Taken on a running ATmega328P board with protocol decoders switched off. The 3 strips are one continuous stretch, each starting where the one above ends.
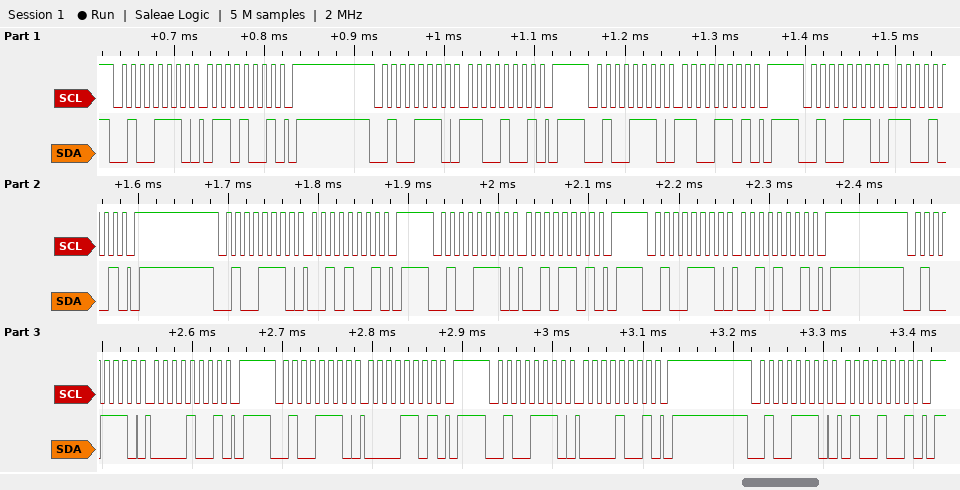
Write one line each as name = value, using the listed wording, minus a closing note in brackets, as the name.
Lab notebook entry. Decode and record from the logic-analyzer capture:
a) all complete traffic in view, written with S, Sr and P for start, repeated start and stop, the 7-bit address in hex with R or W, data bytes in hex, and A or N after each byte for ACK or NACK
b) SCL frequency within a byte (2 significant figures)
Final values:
all complete traffic in view, written with S, Sr and P for start, repeated start and stop, the 7-bit address in hex with R or W, data bytes in hex, and A or N after each byte for ACK or NACK = S 27W A 69 A P S 27W A C9 A P S 27W A CD A P S 27W A C9 A P S 27W A 29 A P S 27W A 2D A P S 27W A 29 A P S 27W A 09 A P S 27W A 0D A P S 27W A 09 A P S 27W A 49 A P
SCL frequency within a byte = 100 kHz
